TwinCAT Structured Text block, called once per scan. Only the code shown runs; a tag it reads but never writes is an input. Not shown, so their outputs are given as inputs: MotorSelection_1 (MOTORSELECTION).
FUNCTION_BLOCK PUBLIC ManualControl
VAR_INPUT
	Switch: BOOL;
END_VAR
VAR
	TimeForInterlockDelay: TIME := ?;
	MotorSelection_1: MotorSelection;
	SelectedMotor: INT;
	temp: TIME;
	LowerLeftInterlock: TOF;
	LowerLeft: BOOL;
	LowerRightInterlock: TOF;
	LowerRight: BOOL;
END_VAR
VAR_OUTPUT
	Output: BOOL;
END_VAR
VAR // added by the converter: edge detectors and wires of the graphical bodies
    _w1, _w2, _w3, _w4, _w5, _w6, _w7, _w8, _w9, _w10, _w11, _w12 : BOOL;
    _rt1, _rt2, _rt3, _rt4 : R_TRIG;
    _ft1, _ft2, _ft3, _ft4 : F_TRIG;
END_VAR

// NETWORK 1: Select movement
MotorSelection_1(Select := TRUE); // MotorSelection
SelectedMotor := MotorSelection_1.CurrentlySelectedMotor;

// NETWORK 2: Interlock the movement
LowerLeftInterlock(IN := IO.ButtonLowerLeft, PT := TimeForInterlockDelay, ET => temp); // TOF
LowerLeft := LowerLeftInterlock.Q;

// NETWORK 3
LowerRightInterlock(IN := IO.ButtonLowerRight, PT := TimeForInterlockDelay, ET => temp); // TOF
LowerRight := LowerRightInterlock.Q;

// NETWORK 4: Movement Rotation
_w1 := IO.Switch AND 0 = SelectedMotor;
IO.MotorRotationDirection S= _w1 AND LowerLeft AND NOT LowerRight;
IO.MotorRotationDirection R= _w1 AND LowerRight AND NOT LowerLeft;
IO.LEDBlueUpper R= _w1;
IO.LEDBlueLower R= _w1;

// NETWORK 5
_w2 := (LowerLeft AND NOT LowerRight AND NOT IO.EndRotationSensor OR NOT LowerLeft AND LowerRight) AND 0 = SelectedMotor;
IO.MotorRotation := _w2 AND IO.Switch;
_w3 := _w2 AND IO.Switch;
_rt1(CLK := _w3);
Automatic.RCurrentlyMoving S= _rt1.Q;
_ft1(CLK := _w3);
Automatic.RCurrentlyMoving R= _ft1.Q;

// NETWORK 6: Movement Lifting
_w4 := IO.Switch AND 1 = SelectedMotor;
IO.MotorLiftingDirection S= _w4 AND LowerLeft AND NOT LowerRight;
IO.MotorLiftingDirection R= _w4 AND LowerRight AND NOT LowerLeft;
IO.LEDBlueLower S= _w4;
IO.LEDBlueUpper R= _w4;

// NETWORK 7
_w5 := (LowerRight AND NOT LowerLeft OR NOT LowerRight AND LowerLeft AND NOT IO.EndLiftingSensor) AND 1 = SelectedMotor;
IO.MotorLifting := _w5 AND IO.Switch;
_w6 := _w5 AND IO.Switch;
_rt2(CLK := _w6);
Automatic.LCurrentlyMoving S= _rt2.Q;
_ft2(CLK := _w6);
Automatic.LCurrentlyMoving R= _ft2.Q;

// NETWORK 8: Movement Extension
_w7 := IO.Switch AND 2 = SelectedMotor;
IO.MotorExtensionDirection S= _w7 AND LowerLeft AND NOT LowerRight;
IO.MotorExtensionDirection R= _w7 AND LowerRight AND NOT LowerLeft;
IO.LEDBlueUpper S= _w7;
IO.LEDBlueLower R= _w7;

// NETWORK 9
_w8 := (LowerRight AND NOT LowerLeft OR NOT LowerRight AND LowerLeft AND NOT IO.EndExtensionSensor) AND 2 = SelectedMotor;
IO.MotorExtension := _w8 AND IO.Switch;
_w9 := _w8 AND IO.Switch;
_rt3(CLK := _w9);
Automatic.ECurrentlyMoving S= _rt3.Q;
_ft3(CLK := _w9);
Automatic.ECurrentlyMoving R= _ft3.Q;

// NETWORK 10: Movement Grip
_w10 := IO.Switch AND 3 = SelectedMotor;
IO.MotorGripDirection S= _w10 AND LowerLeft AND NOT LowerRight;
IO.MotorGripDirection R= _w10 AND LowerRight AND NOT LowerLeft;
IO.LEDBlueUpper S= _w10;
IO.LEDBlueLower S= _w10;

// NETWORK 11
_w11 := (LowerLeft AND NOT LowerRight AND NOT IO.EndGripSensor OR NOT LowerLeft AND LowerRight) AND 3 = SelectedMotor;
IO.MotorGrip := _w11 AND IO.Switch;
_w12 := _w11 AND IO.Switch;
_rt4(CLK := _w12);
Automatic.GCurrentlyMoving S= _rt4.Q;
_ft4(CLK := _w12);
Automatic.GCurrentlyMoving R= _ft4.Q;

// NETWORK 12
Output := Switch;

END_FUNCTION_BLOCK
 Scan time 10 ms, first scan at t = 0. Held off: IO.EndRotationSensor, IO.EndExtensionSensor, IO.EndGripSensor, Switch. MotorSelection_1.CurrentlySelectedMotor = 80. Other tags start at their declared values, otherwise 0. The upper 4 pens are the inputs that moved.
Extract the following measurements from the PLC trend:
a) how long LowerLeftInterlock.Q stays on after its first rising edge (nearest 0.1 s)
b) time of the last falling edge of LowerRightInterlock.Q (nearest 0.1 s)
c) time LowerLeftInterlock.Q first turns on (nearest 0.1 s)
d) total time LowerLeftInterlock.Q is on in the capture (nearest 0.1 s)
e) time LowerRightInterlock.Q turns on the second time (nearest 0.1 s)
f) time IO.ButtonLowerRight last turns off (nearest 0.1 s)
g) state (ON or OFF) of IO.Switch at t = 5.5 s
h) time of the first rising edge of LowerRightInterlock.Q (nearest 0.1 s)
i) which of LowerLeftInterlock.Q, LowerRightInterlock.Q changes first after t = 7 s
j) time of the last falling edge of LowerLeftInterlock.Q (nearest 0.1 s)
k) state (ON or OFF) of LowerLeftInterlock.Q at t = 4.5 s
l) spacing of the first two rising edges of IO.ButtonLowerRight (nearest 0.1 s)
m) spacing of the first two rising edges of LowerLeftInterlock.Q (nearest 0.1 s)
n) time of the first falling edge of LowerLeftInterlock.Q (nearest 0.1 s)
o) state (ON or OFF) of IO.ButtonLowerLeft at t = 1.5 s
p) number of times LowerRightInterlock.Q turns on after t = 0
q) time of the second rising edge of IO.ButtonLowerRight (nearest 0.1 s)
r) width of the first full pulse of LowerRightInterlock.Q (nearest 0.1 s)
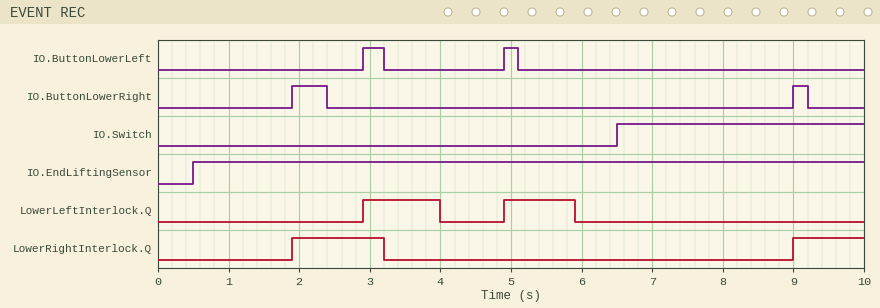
1.1 s
3.2 s
2.9 s
2.1 s
9.0 s
9.2 s
OFF
1.9 s
LowerRightInterlock.Q
5.9 s
OFF
7.1 s
2.0 s
4.0 s
OFF
2
9.0 s
1.3 s
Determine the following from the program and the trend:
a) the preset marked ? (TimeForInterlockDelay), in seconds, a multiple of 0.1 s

0.8 s
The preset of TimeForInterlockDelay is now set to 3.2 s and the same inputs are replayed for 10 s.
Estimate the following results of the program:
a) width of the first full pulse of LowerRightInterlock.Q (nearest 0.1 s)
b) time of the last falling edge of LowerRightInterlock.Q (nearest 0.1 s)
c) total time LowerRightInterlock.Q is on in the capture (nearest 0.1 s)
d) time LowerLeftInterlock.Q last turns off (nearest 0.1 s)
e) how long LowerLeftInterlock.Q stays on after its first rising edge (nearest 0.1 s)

3.7 s
5.6 s
4.7 s
8.3 s
5.4 s
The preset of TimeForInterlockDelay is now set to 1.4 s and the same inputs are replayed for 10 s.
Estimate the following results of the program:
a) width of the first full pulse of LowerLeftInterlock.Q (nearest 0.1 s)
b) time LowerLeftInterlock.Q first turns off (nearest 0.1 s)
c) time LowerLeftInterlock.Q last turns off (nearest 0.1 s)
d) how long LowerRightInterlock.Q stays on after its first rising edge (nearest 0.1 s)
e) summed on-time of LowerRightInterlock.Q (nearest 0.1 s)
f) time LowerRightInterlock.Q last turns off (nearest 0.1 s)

1.7 s
4.6 s
6.5 s
1.9 s
2.9 s
3.8 s
